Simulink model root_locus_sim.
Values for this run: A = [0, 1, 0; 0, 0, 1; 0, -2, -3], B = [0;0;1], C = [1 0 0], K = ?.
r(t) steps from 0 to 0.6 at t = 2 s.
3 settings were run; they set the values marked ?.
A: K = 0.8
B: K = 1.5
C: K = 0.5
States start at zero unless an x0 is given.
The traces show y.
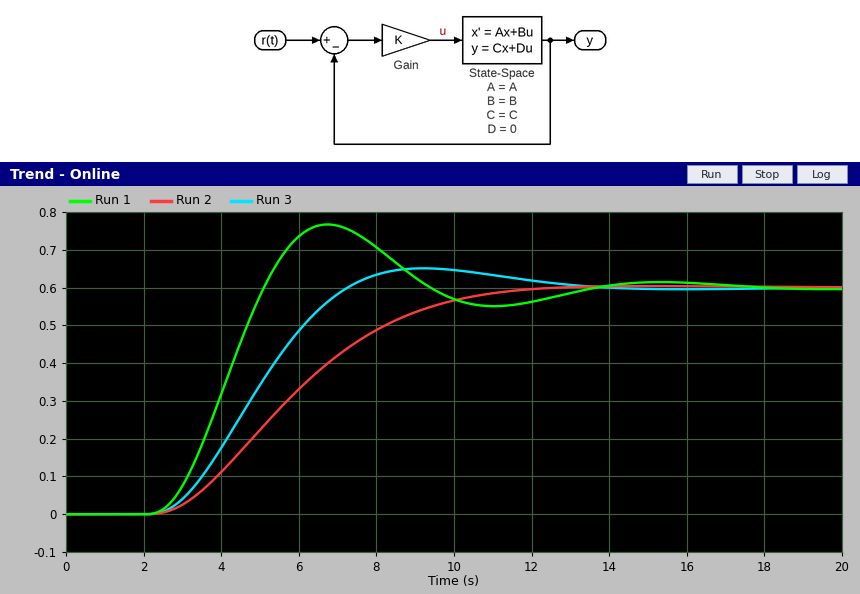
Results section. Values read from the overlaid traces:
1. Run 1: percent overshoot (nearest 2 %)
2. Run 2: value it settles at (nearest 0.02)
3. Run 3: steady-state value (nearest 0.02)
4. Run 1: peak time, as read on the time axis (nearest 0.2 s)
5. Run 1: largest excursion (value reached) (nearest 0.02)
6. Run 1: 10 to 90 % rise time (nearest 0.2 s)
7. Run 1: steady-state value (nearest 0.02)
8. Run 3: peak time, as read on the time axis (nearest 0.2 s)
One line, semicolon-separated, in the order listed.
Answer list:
28 %; 0.60; 0.60; 6.8 s; 0.76; 2.0 s; 0.60; 9.2 s
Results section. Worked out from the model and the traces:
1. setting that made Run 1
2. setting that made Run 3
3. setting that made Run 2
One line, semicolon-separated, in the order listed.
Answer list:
B; A; C
